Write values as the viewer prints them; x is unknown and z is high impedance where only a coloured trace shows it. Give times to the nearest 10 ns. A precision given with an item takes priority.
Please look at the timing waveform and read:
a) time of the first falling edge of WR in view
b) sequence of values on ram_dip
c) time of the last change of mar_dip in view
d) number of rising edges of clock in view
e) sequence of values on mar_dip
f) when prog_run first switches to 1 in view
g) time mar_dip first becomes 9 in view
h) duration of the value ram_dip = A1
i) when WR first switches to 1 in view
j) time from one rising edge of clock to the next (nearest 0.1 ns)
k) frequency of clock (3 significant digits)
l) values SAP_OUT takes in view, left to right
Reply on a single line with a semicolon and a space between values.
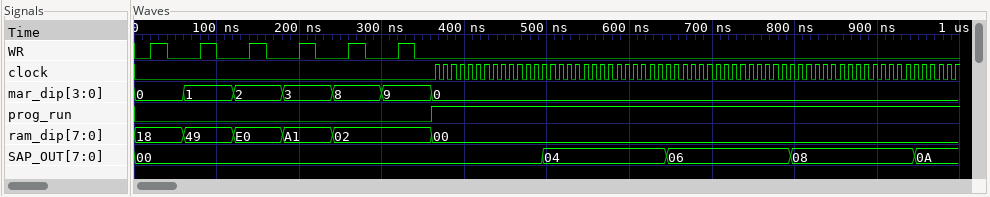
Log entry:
40 ns; 18, 49, E0, A1, 02, 00; 360 ns; 64; 0, 1, 2, 3, 8, 9, 0; 360 ns; 300 ns; 60 ns; 20 ns; 10 ns; 100 MHz; 00, 04, 06, 08, 0A
